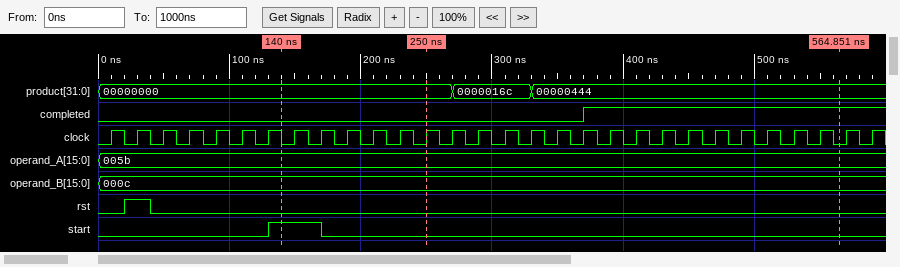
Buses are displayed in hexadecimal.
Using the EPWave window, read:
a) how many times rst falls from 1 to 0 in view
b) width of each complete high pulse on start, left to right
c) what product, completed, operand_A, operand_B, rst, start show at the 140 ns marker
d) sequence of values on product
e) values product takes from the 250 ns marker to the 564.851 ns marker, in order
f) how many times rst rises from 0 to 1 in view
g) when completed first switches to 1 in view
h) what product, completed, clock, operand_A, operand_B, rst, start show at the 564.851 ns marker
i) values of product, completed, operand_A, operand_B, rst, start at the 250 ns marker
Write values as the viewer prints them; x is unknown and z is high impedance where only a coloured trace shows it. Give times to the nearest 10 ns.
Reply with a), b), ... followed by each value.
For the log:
a) 1
b) 40 ns
c) product=00000000, completed=0, operand_A=005b, operand_B=000c, rst=0, start=1
d) 00000000, 0000016c, 00000444
e) 00000000, 0000016c, 00000444
f) 1
g) 370 ns
h) product=00000444, completed=1, clock=0, operand_A=005b, operand_B=000c, rst=0, start=0
i) product=00000000, completed=0, operand_A=005b, operand_B=000c, rst=0, start=0
